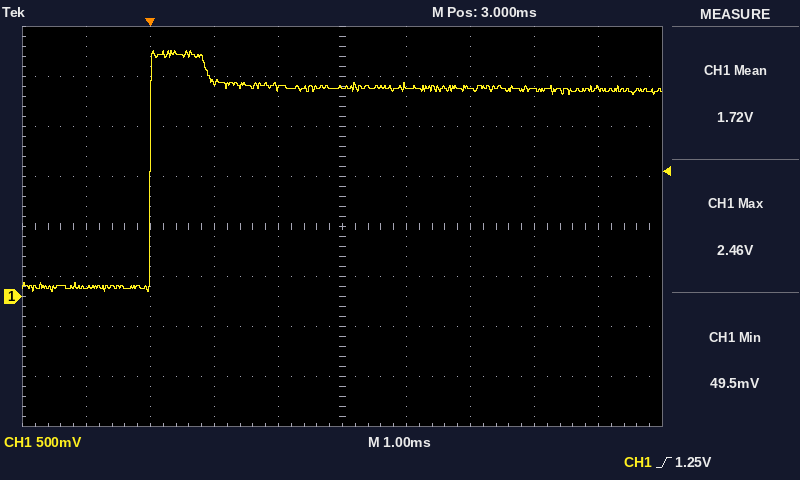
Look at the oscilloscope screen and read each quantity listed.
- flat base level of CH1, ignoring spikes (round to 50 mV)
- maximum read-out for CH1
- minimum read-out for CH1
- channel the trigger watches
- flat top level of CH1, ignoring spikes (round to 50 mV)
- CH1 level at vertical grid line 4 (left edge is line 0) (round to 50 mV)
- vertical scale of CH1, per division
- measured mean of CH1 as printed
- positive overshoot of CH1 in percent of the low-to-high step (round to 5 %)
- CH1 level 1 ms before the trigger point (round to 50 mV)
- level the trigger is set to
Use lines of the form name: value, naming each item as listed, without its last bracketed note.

flat base level of CH1, ignoring spikes: 100 mV
maximum read-out for CH1: 2.46 V
minimum read-out for CH1: 49.5 mV
channel the trigger watches: CH1
flat top level of CH1, ignoring spikes: 2.10 V
CH1 level at vertical grid line 4 (left edge is line 0): 2.10 V
vertical scale of CH1, per division: 500 mV
measured mean of CH1 as printed: 1.72 V
positive overshoot of CH1 in percent of the low-to-high step: 20 %
CH1 level 1 ms before the trigger point: 100 mV
level the trigger is set to: 1.25 V
